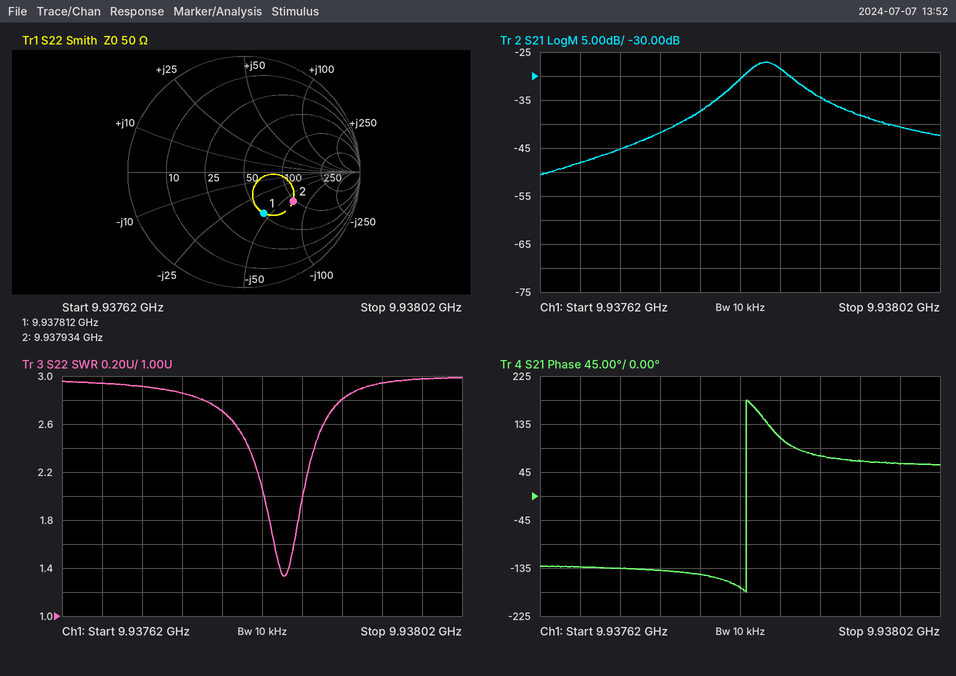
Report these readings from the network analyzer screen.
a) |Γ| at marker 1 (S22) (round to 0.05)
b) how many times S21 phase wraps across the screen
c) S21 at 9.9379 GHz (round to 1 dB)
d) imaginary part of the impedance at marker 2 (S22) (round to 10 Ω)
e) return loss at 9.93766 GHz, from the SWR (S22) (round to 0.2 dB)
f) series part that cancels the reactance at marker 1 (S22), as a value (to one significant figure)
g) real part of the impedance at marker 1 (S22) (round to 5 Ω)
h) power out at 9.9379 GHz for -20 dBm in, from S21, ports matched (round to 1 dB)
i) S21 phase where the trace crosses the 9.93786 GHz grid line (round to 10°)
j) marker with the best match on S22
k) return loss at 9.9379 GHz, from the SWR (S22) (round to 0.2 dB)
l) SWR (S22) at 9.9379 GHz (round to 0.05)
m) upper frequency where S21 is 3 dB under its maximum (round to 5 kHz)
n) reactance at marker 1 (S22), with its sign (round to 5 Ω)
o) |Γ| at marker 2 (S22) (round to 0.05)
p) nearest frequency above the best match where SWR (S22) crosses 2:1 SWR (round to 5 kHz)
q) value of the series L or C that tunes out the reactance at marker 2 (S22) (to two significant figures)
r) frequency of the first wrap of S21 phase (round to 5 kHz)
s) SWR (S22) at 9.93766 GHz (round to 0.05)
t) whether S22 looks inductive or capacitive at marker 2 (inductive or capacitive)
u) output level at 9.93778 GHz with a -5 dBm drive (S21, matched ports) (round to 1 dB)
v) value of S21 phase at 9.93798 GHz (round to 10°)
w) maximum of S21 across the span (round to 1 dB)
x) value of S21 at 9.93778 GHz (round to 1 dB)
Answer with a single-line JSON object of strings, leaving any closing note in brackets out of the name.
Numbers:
{"|Γ| at marker 1 (S22)": "0.40", "how many times S21 phase wraps across the screen": "1", "S21 at 9.9379 GHz": "-34 dB", "imaginary part of the impedance at marker 2 (S22)": "-60 Ω", "return loss at 9.93766 GHz, from the SWR (S22)": "6.2 dB", "series part that cancels the reactance at marker 1 (S22), as a value": "700 pH", "real part of the impedance at marker 1 (S22)": "50 Ω", "power out at 9.9379 GHz for -20 dBm in, from S21, ports matched": "-54 dBm", "S21 phase where the trace crosses the 9.93786 GHz grid line": "110°", "marker with the best match on S22": "marker 1", "return loss at 9.9379 GHz, from the SWR (S22)": "6.4 dB", "SWR (S22) at 9.9379 GHz": "2.80", "upper frequency where S21 is 3 dB under its maximum": "9.937870 GHz", "reactance at marker 1 (S22), with its sign": "-45 Ω", "|Γ| at marker 2 (S22)": "0.50", "nearest frequency above the best match where SWR (S22) crosses 2:1 SWR": "9.937860 GHz", "value of the series L or C that tunes out the reactance at marker 2 (S22)": "1.0 nH", "frequency of the first wrap of S21 phase": "9.937825 GHz", "SWR (S22) at 9.93766 GHz": "2.95", "whether S22 looks inductive or capacitive at marker 2": "capacitive", "output level at 9.93778 GHz with a -5 dBm drive (S21, matched ports)": "-42 dBm", "value of S21 phase at 9.93798 GHz": "60°", "maximum of S21 across the span": "-27 dB", "value of S21 at 9.93778 GHz": "-37 dB"}
